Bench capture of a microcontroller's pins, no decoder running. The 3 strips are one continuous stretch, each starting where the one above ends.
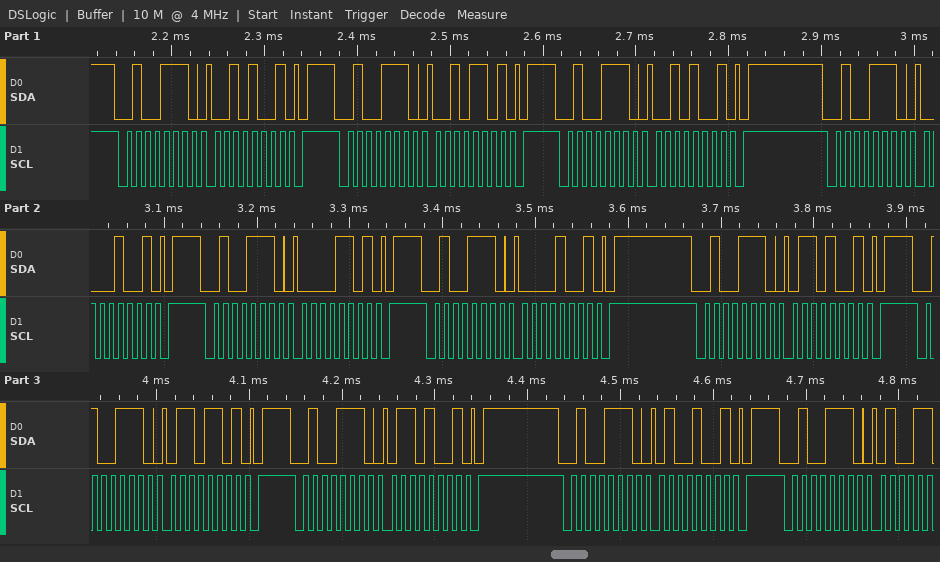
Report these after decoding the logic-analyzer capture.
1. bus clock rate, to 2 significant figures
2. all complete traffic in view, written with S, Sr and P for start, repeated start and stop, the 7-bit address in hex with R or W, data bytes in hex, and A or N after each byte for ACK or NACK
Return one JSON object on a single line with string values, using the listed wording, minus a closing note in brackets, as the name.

{"bus clock rate, to 2 significant figures": "100 kHz", "all complete traffic in view, written with S, Sr and P for start, repeated start and stop, the 7-bit address in hex with R or W, data bytes in hex, and A or N after each byte for ACK or NACK": "S 27W A 29 A P S 27W A 2D A P S 27W A 29 A P S 27W A 09 A P S 27W A 0D A P S 27W A 09 A P S 27W A 69 A P S 27W A 6D A P S 27W A 69 A P S 27W A 49 A P S 27W A"}
